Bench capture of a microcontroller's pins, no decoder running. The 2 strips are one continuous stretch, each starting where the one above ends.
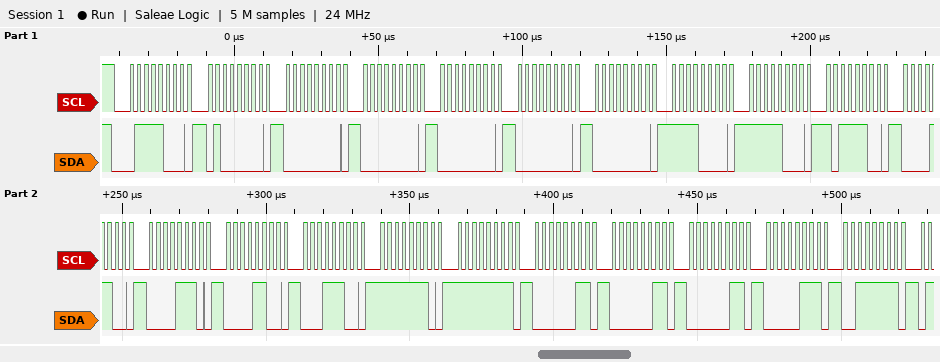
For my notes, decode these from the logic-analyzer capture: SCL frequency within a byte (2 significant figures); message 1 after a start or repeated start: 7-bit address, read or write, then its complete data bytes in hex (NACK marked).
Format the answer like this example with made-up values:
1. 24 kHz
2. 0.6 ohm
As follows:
1. 400 kHz
2. 0x3C write: 40 00 00 00 00 00 F0 F8 BC 0C 0E 0C 1C FE FF 03 03 03 07 3F
